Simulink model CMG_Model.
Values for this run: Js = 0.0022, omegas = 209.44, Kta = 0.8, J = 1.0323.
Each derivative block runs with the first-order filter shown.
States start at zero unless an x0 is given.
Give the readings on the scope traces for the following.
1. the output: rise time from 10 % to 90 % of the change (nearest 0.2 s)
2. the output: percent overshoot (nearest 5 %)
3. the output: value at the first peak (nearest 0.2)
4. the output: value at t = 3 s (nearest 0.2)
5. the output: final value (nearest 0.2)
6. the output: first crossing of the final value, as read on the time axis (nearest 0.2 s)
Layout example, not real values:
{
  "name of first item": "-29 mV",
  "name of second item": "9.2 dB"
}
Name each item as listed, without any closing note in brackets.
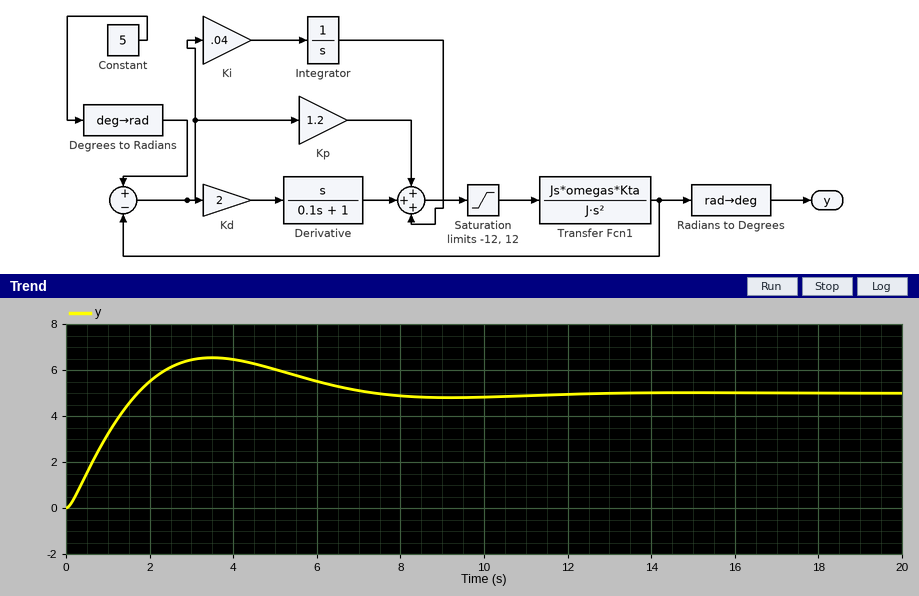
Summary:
{
  "the output: rise time from 10 % to 90 % of the change": "1.2 s",
  "the output: percent overshoot": "30 %",
  "the output: value at the first peak": "6.6",
  "the output: value at t = 3 s": "6.4",
  "the output: final value": "5.0",
  "the output: first crossing of the final value, as read on the time axis": "1.8 s"
}
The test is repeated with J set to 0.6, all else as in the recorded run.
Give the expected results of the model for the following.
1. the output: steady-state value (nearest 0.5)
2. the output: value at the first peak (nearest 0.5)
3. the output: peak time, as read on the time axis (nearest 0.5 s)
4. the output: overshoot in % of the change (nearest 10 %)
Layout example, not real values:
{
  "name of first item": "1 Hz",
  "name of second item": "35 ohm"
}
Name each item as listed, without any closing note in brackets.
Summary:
{
  "the output: steady-state value": "5.0",
  "the output: value at the first peak": "6.0",
  "the output: peak time, as read on the time axis": "2.5 s",
  "the output: overshoot in % of the change": "20 %"
}
